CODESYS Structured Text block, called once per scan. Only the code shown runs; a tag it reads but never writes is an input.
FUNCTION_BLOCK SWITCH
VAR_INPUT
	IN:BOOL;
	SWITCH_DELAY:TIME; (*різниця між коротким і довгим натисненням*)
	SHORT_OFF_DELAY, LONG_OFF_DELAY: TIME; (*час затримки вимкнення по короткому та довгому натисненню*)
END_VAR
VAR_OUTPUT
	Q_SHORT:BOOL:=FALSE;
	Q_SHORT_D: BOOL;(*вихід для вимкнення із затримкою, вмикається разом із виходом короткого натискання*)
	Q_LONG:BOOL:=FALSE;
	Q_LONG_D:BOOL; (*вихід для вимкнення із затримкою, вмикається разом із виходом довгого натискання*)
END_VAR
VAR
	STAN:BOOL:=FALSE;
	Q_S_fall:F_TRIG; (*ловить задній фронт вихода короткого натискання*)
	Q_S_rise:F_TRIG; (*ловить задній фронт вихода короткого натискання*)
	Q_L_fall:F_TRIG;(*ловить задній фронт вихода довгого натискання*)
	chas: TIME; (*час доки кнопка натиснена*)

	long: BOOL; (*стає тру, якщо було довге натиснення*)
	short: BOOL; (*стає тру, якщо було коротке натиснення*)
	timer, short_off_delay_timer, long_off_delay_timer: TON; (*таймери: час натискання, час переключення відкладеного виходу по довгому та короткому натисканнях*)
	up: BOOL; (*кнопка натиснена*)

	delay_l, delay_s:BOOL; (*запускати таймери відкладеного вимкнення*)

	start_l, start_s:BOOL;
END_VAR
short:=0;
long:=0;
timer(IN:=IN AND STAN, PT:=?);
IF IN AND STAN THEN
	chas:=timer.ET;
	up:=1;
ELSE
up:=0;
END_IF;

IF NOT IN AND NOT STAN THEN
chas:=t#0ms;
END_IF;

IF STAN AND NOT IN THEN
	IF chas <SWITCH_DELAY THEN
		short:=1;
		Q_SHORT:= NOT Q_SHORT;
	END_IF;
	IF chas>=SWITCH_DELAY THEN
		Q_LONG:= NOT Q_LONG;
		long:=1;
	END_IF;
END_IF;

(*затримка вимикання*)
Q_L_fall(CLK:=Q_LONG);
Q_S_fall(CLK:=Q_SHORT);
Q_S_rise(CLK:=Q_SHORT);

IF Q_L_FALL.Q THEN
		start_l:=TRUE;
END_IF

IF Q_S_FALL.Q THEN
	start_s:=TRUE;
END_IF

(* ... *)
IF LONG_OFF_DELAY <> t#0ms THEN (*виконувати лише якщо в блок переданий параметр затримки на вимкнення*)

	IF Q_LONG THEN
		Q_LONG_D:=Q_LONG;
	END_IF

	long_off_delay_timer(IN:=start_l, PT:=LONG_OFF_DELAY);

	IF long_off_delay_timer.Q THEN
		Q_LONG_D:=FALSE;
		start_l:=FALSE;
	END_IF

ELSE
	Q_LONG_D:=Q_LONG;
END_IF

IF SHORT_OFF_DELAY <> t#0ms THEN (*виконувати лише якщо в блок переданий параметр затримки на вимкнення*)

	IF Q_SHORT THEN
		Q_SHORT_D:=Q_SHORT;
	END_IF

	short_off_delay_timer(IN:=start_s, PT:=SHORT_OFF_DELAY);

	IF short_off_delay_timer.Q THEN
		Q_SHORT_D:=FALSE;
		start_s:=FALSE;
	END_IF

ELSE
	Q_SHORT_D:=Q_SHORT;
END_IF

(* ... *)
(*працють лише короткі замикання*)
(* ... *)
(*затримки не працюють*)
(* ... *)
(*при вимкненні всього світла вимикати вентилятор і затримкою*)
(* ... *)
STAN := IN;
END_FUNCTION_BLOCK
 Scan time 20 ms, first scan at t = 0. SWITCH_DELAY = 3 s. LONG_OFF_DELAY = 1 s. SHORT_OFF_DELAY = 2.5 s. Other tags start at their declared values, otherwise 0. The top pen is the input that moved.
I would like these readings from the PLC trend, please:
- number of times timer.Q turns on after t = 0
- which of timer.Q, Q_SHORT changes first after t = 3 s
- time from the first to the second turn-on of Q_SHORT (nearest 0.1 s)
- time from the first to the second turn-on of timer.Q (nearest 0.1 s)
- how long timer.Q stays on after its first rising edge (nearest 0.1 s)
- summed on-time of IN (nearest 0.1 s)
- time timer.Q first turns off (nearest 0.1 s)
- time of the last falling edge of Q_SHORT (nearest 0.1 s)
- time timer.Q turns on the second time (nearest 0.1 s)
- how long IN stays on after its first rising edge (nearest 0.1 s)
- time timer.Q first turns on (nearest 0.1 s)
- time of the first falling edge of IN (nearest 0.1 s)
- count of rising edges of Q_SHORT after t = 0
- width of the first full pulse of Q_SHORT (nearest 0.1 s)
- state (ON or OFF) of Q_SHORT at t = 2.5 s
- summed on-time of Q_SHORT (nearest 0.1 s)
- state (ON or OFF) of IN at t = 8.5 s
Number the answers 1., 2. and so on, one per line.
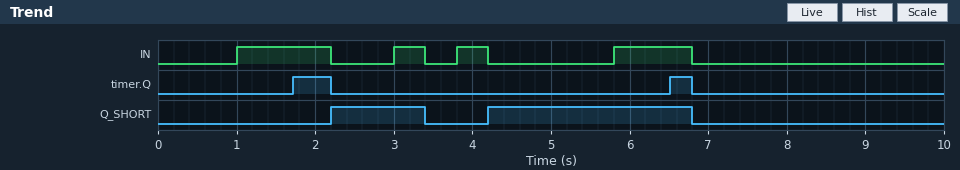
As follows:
1. 2
2. Q_SHORT
3. 2.0 s
4. 4.8 s
5. 0.5 s
6. 3.0 s
7. 2.2 s
8. 6.8 s
9. 6.5 s
10. 1.2 s
11. 1.7 s
12. 2.2 s
13. 2
14. 1.2 s
15. ON
16. 3.8 s
17. OFF
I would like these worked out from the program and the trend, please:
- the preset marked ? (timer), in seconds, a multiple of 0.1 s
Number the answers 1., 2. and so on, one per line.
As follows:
1. 0.7 s
